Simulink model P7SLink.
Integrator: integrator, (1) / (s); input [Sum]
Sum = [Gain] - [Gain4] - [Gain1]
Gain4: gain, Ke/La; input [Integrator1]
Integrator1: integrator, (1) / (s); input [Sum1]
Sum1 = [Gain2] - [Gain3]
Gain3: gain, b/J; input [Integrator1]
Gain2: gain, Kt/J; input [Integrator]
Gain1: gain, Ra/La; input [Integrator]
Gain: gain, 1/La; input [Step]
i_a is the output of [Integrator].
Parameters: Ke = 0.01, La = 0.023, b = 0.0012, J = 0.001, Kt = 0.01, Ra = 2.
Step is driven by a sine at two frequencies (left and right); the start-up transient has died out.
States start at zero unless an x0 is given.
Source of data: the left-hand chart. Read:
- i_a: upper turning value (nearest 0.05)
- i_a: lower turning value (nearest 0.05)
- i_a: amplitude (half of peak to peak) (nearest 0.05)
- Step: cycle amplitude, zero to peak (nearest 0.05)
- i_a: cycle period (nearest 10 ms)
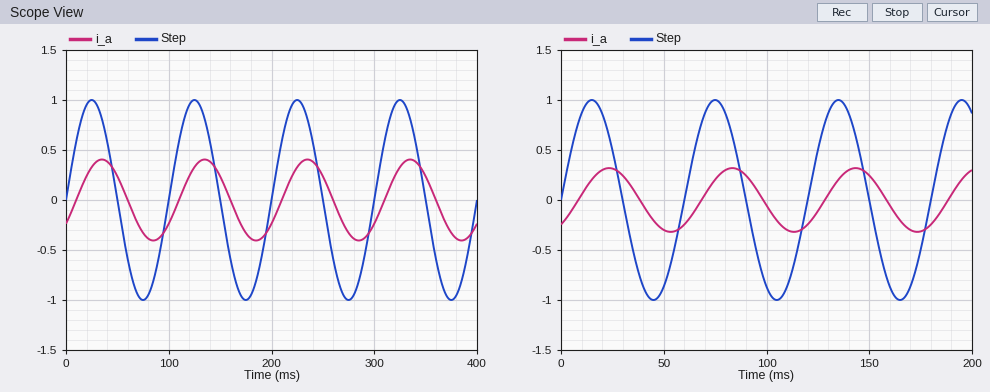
0.40
-0.40
0.40
1.00
100 ms
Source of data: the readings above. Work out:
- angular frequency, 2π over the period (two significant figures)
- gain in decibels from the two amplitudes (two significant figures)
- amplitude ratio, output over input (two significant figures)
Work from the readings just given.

0.063 rad/ms
-8.0 dB
0.40
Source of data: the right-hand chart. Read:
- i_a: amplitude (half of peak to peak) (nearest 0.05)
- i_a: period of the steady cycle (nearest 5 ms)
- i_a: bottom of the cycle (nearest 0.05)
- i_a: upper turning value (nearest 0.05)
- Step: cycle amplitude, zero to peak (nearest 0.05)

0.30
60 ms
-0.30
0.30
1.00
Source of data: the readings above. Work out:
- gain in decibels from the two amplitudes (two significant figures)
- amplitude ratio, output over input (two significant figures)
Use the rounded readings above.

-10 dB
0.30
